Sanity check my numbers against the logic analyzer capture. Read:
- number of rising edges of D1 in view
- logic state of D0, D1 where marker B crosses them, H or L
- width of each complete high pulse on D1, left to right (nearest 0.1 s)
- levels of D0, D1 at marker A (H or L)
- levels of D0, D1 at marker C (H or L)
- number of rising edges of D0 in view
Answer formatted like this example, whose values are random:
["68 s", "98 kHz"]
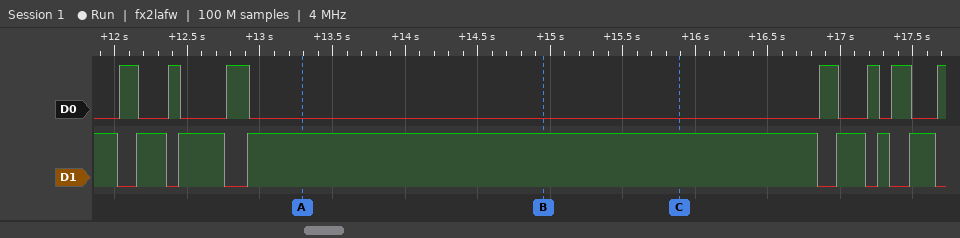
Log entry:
["6", "D0=L, D1=H", "0.2 s, 0.3 s, 3.9 s, 0.2 s, 0.1 s, 0.2 s", "D0=L, D1=H", "D0=L, D1=H", "7"]
